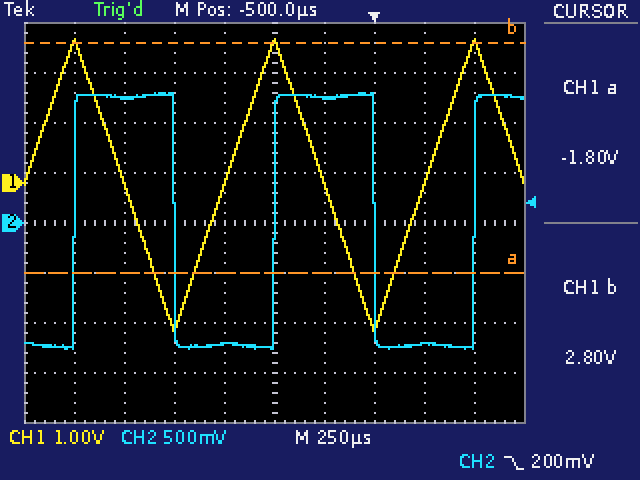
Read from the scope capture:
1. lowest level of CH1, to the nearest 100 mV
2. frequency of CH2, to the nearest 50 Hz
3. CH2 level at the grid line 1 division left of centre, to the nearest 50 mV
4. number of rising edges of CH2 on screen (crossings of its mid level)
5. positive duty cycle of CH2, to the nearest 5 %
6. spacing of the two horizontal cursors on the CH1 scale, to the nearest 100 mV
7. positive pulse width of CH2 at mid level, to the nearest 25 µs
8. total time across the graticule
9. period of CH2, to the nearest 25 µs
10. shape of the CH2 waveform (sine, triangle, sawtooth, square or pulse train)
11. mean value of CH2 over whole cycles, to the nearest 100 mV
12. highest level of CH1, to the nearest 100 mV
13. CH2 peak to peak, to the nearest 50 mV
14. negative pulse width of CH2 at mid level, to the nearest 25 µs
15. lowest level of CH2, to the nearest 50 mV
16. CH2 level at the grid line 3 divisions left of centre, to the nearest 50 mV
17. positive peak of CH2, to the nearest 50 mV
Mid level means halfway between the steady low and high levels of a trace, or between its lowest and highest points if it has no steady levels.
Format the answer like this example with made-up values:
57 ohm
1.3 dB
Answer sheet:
-3.0 V
1.00 kHz
-1.20 V
3
50 %
4.6 V
500 µs
2.5 ms
1.000 ms
square
0.0 V
2.9 V
2.55 V
500 µs
-1.25 V
1.25 V
1.30 V
